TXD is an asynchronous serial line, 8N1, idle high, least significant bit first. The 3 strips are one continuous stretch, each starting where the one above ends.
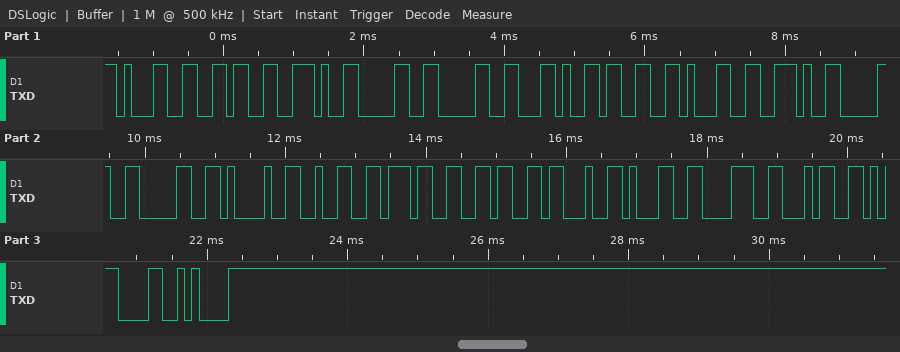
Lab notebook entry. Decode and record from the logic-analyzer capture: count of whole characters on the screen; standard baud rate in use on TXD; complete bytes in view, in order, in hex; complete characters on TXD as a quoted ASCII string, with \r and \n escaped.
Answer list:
21
9600 baud
31 36 2E 30 30 2C 33 31 2E 30 30 21 32 37 36 23 31 38 34 0D 0A
"16.00,31.00!276#184\r\n"
